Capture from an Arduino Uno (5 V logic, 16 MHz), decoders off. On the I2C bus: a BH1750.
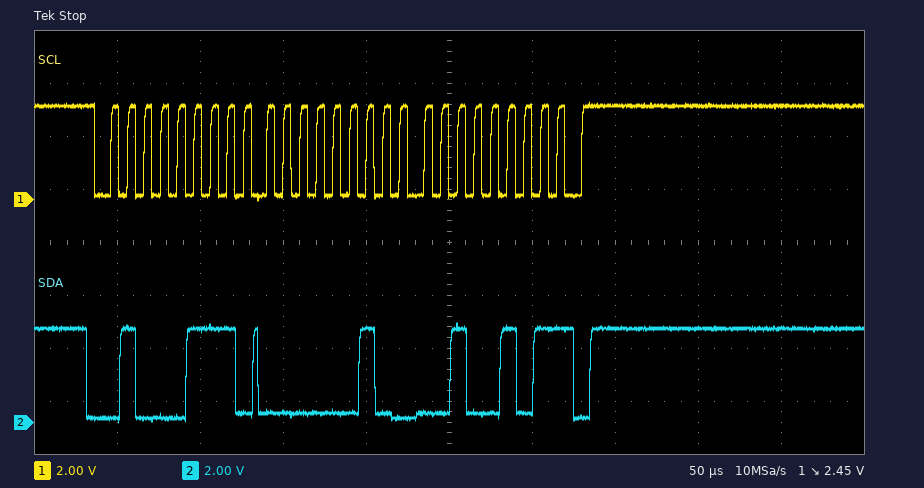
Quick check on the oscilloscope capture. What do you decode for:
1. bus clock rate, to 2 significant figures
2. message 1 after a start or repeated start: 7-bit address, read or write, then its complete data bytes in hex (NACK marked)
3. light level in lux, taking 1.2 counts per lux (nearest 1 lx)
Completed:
100 kHz
0x23 read: 02 25 NACK
458 lx
